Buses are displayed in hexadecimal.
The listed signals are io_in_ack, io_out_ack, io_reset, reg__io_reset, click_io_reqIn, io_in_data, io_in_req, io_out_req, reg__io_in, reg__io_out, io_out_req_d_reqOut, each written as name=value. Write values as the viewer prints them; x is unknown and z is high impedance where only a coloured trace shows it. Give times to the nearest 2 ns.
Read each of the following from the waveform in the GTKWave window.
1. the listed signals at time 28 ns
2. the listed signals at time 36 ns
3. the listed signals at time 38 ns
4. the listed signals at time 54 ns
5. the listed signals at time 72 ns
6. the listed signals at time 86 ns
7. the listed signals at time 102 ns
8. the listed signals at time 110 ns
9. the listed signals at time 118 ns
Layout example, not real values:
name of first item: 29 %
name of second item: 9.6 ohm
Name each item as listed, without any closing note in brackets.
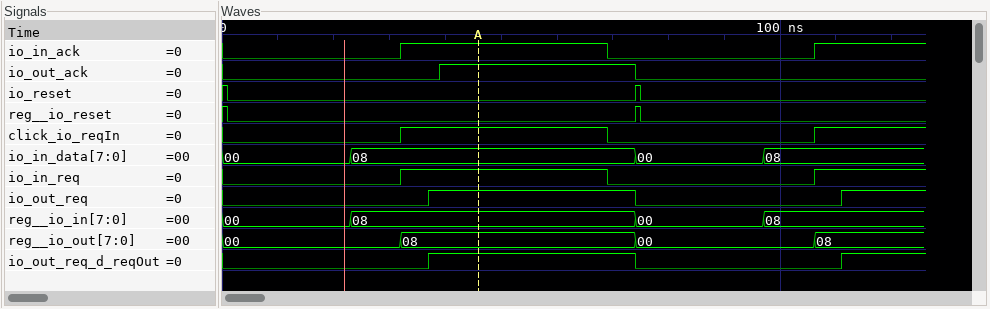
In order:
the listed signals at time 28 ns: io_in_ack=0, io_out_ack=0, io_reset=0, reg__io_reset=0, click_io_reqIn=0, io_in_data=08, io_in_req=0, io_out_req=0, reg__io_in=08, reg__io_out=00, io_out_req_d_reqOut=0
the listed signals at time 36 ns: io_in_ack=1, io_out_ack=0, io_reset=0, reg__io_reset=0, click_io_reqIn=1, io_in_data=08, io_in_req=1, io_out_req=0, reg__io_in=08, reg__io_out=08, io_out_req_d_reqOut=0
the listed signals at time 38 ns: io_in_ack=1, io_out_ack=0, io_reset=0, reg__io_reset=0, click_io_reqIn=1, io_in_data=08, io_in_req=1, io_out_req=1, reg__io_in=08, reg__io_out=08, io_out_req_d_reqOut=1
the listed signals at time 54 ns: io_in_ack=1, io_out_ack=1, io_reset=0, reg__io_reset=0, click_io_reqIn=1, io_in_data=08, io_in_req=1, io_out_req=1, reg__io_in=08, reg__io_out=08, io_out_req_d_reqOut=1
the listed signals at time 72 ns: io_in_ack=0, io_out_ack=1, io_reset=0, reg__io_reset=0, click_io_reqIn=0, io_in_data=08, io_in_req=0, io_out_req=1, reg__io_in=08, reg__io_out=08, io_out_req_d_reqOut=1
the listed signals at time 86 ns: io_in_ack=0, io_out_ack=0, io_reset=0, reg__io_reset=0, click_io_reqIn=0, io_in_data=00, io_in_req=0, io_out_req=0, reg__io_in=00, reg__io_out=00, io_out_req_d_reqOut=0
the listed signals at time 102 ns: io_in_ack=0, io_out_ack=0, io_reset=0, reg__io_reset=0, click_io_reqIn=0, io_in_data=08, io_in_req=0, io_out_req=0, reg__io_in=08, reg__io_out=00, io_out_req_d_reqOut=0
the listed signals at time 110 ns: io_in_ack=1, io_out_ack=0, io_reset=0, reg__io_reset=0, click_io_reqIn=1, io_in_data=08, io_in_req=1, io_out_req=0, reg__io_in=08, reg__io_out=08, io_out_req_d_reqOut=0
the listed signals at time 118 ns: io_in_ack=1, io_out_ack=0, io_reset=0, reg__io_reset=0, click_io_reqIn=1, io_in_data=08, io_in_req=1, io_out_req=1, reg__io_in=08, reg__io_out=08, io_out_req_d_reqOut=1
